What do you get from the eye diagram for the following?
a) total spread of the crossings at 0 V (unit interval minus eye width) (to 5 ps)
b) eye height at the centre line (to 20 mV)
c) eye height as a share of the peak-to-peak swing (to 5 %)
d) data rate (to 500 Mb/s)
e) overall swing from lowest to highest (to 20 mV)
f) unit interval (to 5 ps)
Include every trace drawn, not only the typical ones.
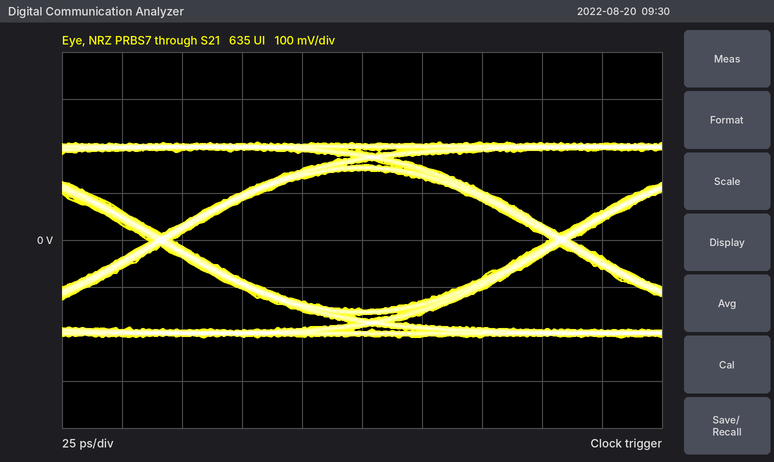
10 ps
300 mV
70 %
6.0 Gb/s
420 mV
165 ps
